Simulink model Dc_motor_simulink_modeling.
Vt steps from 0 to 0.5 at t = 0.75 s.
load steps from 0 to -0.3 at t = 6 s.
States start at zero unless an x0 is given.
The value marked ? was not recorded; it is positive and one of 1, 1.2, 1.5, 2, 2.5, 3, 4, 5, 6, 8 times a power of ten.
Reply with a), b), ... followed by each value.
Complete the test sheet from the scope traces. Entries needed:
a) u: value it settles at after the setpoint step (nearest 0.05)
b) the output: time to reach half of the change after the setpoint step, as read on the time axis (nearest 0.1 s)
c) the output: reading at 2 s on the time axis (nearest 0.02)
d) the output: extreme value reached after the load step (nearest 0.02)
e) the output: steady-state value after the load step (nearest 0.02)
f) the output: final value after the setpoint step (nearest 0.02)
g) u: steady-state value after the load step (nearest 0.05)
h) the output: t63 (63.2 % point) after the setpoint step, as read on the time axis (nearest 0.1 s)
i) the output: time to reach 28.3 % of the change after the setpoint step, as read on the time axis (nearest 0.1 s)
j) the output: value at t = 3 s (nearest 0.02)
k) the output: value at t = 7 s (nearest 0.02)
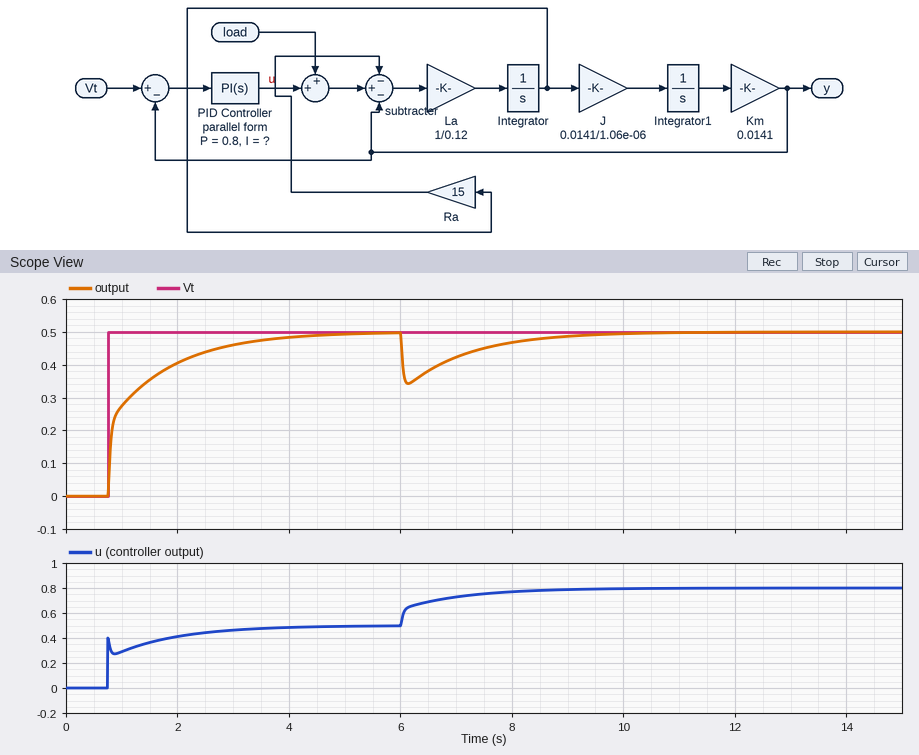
a) 0.50
b) 0.9 s
c) 0.40
d) 0.34
e) 0.50
f) 0.50
g) 0.80
h) 1.2 s
i) 0.8 s
j) 0.46
k) 0.42
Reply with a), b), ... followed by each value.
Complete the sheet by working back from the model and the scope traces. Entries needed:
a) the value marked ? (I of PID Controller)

a) 1.5
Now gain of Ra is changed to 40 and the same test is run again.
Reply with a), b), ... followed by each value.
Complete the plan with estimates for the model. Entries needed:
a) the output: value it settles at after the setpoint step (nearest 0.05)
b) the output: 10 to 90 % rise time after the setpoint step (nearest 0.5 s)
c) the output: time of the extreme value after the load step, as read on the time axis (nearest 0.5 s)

a) 0.50
b) 2.0 s
c) 6.5 s
